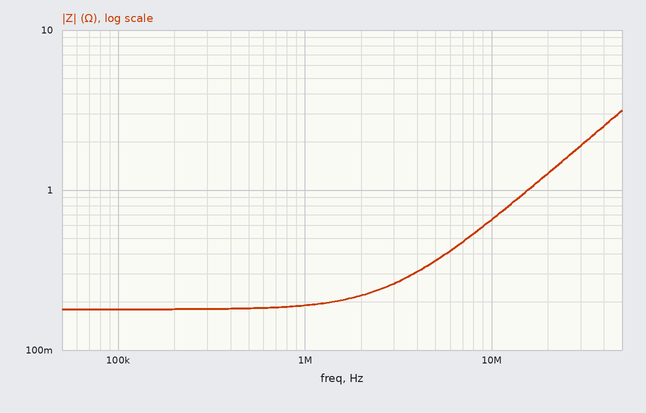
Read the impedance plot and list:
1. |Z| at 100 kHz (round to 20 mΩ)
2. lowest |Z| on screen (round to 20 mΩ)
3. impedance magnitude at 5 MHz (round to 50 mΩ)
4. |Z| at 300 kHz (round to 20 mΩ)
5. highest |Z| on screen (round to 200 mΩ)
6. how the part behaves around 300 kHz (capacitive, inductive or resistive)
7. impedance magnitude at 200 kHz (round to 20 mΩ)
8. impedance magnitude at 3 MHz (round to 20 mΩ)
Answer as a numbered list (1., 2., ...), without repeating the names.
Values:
1. 180 mΩ
2. 180 mΩ
3. 350 mΩ
4. 180 mΩ
5. 3.2 Ω
6. resistive
7. 180 mΩ
8. 260 mΩ
